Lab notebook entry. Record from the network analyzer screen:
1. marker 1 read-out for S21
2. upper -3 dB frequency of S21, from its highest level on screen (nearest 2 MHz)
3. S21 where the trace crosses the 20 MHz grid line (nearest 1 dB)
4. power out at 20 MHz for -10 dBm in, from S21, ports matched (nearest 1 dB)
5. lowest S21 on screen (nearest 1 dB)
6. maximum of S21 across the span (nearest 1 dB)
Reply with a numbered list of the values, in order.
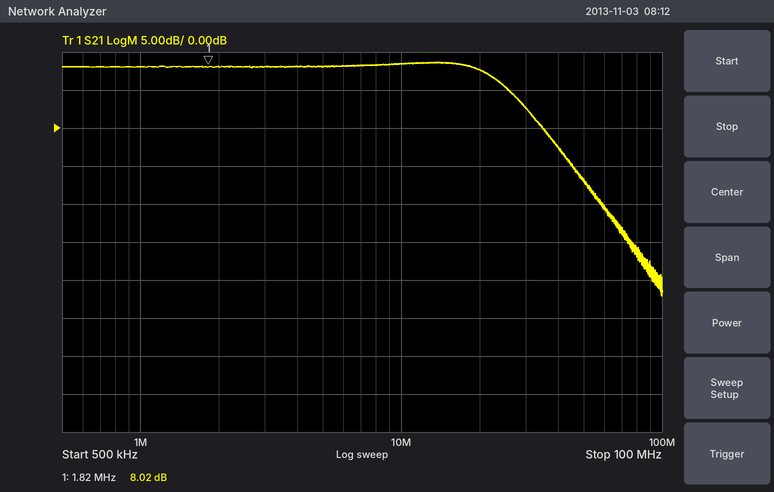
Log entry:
1. 8.02 dB
2. 24 MHz
3. 8 dB
4. -2 dBm
5. -22 dB
6. 9 dB
